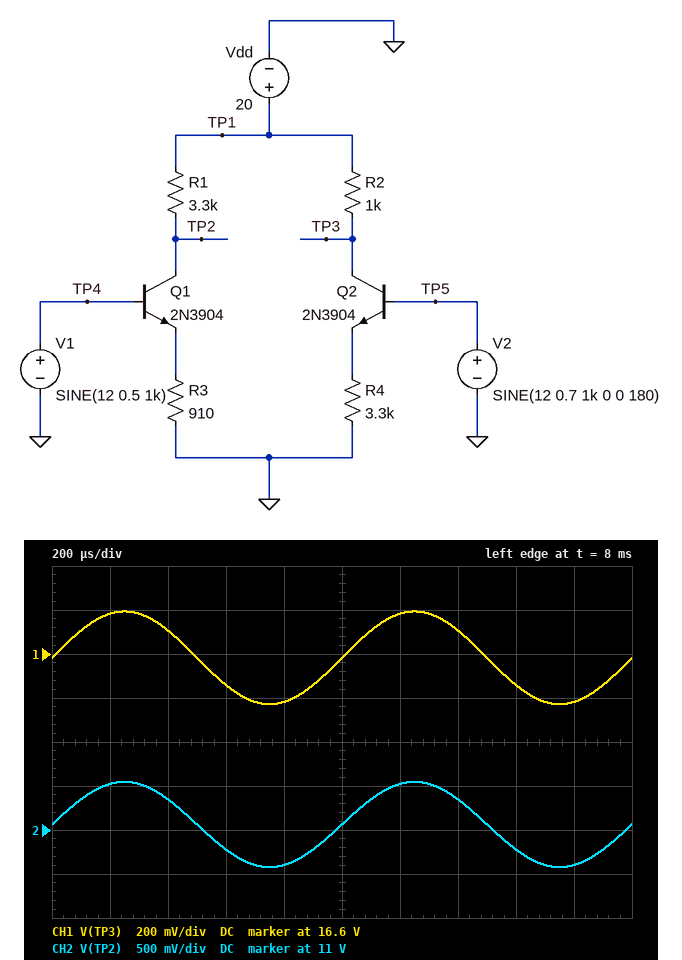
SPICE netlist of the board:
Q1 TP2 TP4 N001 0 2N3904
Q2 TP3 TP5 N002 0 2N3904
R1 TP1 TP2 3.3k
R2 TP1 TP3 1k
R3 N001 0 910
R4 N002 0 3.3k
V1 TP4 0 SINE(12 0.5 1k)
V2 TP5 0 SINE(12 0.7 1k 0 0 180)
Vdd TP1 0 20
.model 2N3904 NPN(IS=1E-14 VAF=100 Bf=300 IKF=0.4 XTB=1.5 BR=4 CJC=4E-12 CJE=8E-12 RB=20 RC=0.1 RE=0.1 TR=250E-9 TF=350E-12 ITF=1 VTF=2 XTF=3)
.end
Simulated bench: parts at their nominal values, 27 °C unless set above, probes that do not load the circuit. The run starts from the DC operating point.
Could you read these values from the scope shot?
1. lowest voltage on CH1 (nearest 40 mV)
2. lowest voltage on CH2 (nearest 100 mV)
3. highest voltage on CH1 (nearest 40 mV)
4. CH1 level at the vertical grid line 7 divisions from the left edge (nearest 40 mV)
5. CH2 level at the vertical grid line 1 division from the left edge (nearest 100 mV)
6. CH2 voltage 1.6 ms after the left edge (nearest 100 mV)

16.36 V
10.6 V
16.80 V
16.72 V
11.5 V
10.8 V
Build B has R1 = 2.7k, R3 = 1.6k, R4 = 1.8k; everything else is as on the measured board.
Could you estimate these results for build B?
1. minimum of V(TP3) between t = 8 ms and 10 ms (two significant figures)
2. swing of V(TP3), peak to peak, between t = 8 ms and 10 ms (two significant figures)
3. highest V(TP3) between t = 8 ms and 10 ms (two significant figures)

13 V
770 mV
14 V
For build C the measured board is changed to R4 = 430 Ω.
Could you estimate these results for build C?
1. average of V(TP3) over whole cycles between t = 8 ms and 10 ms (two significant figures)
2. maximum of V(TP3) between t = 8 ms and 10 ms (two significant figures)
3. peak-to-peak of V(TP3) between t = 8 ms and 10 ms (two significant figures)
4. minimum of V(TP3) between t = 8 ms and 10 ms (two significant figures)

11 V
12 V
1.3 V
10 V
